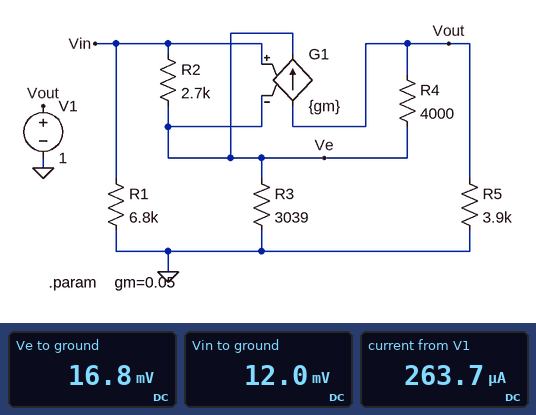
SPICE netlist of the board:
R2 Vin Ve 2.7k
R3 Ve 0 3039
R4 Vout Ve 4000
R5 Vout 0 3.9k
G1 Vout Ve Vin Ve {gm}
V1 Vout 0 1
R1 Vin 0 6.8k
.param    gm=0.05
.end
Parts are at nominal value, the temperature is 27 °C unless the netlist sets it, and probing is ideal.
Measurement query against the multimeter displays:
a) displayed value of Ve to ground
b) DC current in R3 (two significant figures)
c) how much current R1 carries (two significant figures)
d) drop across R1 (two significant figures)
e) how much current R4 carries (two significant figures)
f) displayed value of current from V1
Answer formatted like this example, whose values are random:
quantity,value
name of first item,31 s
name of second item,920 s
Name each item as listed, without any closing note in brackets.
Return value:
quantity,value
displayed value of Ve to ground,16.8 mV
DC current in R3,5.5 µA
how much current R1 carries,1.8 µA
drop across R1,12 mV
how much current R4 carries,250 µA
displayed value of current from V1,263.7 µA
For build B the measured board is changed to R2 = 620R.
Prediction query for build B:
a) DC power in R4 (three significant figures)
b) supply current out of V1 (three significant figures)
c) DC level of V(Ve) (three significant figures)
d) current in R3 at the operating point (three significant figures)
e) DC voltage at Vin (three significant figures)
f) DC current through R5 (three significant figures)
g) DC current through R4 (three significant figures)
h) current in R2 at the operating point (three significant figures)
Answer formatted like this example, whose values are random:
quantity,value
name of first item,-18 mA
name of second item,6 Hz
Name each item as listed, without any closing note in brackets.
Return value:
quantity,value
DC power in R4,225 µW
supply current out of V1,280 µA
DC level of V(Ve),51.1 mV
current in R3 at the operating point,16.8 µA
DC voltage at Vin,46.8 mV
DC current through R5,256 µA
DC current through R4,237 µA
current in R2 at the operating point,6.89 µA
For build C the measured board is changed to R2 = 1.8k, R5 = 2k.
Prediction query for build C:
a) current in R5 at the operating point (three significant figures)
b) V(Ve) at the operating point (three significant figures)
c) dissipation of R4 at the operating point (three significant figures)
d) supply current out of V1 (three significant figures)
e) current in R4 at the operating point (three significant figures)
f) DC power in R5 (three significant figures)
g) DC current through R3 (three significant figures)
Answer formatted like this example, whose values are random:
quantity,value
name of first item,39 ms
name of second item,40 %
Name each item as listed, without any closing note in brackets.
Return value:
quantity,value
current in R5 at the operating point,500 µA
V(Ve) at the operating point,22.4 mV
dissipation of R4 at the operating point,239 µW
supply current out of V1,510 µA
current in R4 at the operating point,244 µA
DC power in R5,500 µW
DC current through R3,7.37 µA
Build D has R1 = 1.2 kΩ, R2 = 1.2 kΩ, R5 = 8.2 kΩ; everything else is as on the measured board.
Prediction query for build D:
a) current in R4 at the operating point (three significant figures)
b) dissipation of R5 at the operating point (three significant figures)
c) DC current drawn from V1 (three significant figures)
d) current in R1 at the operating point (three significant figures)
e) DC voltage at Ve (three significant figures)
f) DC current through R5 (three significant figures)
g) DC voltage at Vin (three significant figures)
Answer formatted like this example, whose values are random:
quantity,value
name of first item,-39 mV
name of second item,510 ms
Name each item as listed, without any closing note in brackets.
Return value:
quantity,value
current in R4 at the operating point,248 µA
dissipation of R5 at the operating point,122 µW
DC current drawn from V1,129 µA
current in R1 at the operating point,4.01 µA
DC voltage at Ve,9.62 mV
DC current through R5,122 µA
DC voltage at Vin,4.81 mV
